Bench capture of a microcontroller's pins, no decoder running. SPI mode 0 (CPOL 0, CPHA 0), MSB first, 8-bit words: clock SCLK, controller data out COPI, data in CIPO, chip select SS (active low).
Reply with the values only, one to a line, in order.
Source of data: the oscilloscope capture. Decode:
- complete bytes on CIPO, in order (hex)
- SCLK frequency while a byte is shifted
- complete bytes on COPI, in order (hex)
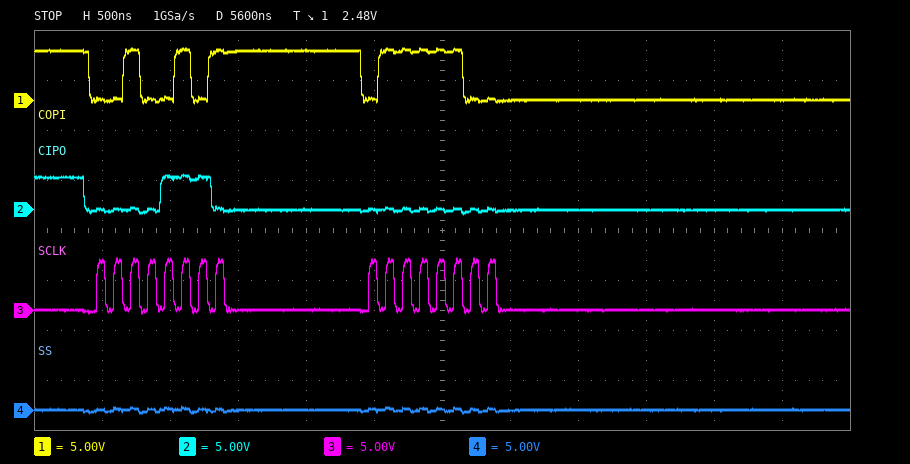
0E 00
8 MHz
25 7C
